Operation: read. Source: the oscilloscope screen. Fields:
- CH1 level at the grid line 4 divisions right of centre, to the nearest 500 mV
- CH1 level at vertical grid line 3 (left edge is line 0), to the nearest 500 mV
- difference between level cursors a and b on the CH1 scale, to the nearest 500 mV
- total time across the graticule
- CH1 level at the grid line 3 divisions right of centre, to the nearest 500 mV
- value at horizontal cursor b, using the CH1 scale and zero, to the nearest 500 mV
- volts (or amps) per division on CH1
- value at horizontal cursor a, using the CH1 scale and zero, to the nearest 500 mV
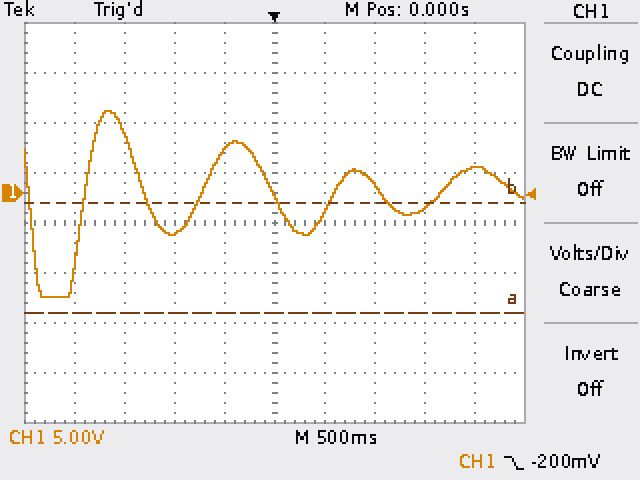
2.5 V
-4.0 V
11.0 V
5 s
-1.5 V
-1.0 V
5 V
-12.0 V
